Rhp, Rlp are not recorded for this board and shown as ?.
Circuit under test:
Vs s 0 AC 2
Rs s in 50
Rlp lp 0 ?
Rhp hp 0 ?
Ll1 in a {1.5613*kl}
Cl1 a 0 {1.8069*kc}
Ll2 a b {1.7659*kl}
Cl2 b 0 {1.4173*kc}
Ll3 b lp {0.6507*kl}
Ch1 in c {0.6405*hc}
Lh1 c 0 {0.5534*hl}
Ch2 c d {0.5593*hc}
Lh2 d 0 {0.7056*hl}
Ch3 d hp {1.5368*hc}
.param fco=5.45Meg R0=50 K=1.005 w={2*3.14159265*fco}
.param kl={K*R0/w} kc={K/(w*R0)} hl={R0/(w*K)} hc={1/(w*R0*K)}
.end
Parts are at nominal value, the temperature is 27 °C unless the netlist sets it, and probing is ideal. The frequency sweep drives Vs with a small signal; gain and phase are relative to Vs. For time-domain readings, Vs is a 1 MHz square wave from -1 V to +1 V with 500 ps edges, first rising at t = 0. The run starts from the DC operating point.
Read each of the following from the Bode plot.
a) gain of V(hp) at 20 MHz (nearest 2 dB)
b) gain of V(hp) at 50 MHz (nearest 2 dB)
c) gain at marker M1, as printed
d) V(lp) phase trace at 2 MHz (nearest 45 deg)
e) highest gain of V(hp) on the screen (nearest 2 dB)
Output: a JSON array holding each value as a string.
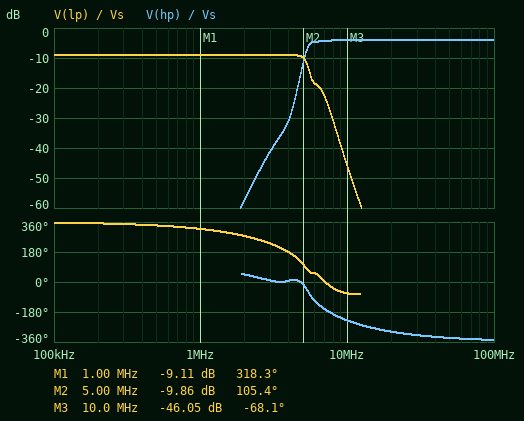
["-4 dB", "-4 dB", "-9.11 dB", "270 deg", "-4 dB"]
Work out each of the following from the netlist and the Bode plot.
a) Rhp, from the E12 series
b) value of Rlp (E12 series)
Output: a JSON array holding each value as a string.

["82 Ω", "27 Ω"]
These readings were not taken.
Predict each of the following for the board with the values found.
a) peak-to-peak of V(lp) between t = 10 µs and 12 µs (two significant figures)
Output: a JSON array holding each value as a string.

["930 mV"]
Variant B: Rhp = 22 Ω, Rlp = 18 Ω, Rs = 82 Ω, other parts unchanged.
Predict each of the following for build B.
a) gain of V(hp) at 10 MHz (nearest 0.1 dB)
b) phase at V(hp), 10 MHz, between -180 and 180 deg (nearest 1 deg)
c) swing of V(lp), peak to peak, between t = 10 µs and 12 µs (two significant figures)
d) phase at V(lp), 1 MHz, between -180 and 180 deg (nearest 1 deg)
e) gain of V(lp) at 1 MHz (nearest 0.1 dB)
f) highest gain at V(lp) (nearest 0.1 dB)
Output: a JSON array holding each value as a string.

["-12.6 dB", "135 deg", "570 mV", "-35 deg", "-14.1 dB", "-12.9 dB"]
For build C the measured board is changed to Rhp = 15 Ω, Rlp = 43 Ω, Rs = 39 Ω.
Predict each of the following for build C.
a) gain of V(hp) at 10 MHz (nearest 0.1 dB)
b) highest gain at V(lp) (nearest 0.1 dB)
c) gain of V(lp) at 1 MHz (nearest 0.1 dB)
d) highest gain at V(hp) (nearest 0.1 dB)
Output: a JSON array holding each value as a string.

["-11.9 dB", "-5.6 dB", "-5.7 dB", "-11.1 dB"]
